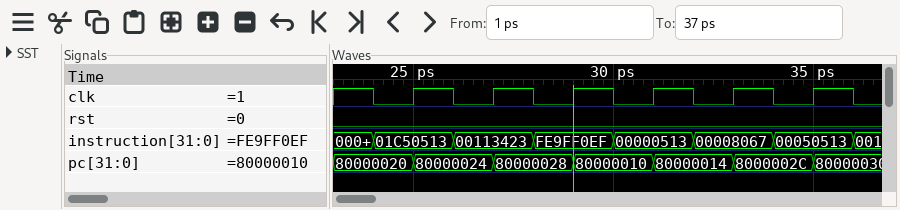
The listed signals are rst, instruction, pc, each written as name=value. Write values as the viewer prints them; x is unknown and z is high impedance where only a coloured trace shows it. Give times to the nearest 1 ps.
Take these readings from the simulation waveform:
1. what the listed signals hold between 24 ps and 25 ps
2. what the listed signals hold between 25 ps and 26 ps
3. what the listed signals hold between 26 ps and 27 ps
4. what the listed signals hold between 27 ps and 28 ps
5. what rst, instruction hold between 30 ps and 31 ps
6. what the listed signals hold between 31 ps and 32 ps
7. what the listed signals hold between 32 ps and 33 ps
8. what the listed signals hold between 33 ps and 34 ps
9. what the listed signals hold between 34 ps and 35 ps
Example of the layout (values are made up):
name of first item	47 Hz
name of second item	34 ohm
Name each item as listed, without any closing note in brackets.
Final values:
what the listed signals hold between 24 ps and 25 ps	rst=0, instruction=01C50513, pc=80000020
what the listed signals hold between 25 ps and 26 ps	rst=0, instruction=01C50513, pc=80000024
what the listed signals hold between 26 ps and 27 ps	rst=0, instruction=00113423, pc=80000024
what the listed signals hold between 27 ps and 28 ps	rst=0, instruction=00113423, pc=80000028
what rst, instruction hold between 30 ps and 31 ps	rst=0, instruction=00000513
what the listed signals hold between 31 ps and 32 ps	rst=0, instruction=00000513, pc=80000014
what the listed signals hold between 32 ps and 33 ps	rst=0, instruction=00008067, pc=80000014
what the listed signals hold between 33 ps and 34 ps	rst=0, instruction=00008067, pc=8000002C
what the listed signals hold between 34 ps and 35 ps	rst=0, instruction=00050513, pc=8000002C
